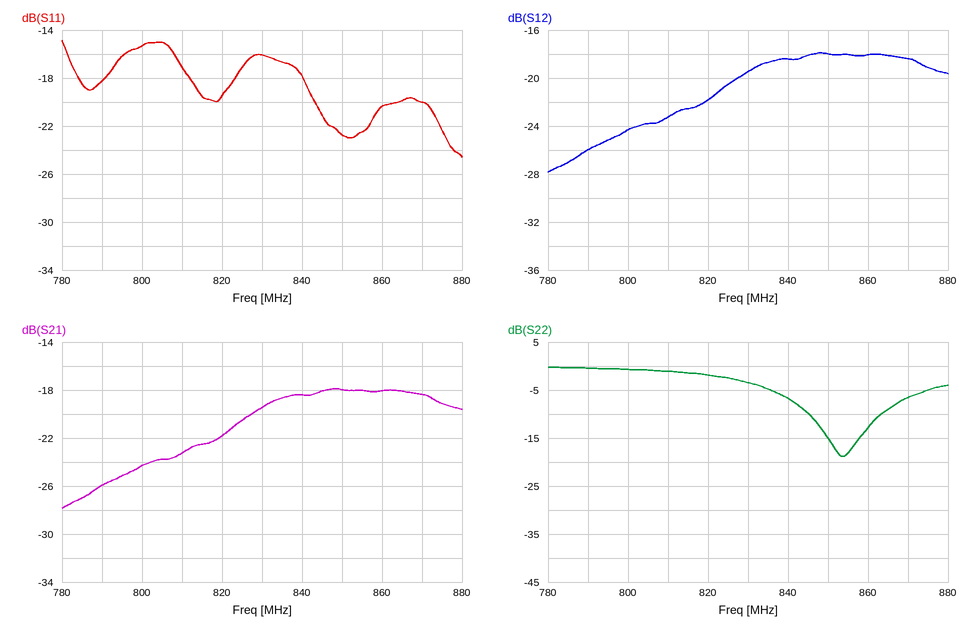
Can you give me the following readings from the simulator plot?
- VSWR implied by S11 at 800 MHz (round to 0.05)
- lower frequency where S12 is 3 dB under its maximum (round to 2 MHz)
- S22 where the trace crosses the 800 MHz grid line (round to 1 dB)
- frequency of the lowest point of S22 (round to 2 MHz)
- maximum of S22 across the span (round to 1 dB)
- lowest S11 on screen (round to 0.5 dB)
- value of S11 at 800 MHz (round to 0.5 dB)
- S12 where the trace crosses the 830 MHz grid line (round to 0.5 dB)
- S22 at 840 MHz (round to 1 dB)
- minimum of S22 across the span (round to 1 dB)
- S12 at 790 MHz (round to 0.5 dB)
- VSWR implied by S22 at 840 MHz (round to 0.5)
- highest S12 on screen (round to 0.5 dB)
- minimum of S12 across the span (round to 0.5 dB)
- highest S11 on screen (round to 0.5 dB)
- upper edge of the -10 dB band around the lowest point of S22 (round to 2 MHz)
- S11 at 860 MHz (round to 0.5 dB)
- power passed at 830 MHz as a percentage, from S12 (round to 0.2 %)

1.40
824 MHz
-1 dB
854 MHz
0 dB
-24.5 dB
-15.5 dB
-19.5 dB
-7 dB
-19 dB
-26.0 dB
2.5
-18.0 dB
-28.0 dB
-15.0 dB
864 MHz
-20.5 dB
1.2 %
